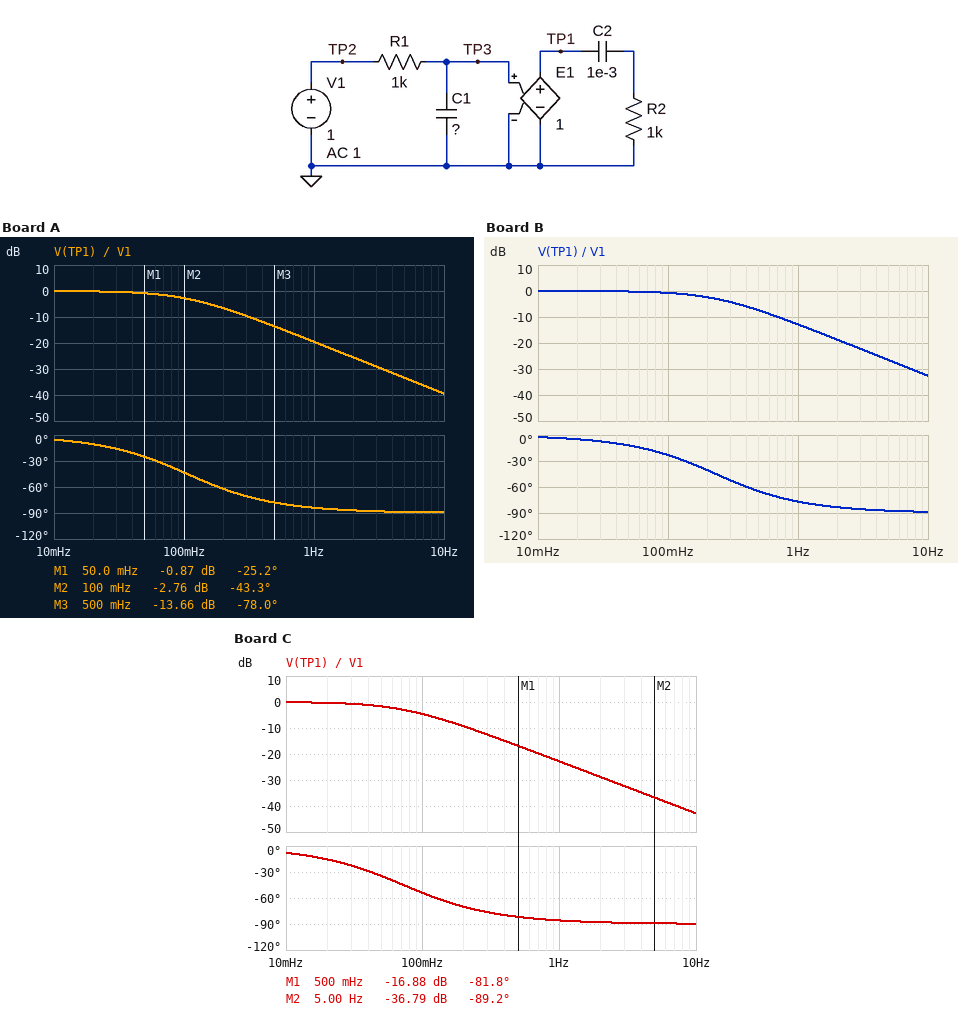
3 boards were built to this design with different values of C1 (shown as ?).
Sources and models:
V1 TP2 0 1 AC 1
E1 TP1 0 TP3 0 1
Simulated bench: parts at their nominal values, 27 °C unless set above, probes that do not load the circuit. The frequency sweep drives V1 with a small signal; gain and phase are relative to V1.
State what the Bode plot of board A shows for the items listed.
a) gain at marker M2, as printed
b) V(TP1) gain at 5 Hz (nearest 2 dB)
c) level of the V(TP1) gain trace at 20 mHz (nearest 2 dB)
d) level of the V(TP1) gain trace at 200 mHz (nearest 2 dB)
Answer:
-2.76 dB
-34 dB
0 dB
-6 dB
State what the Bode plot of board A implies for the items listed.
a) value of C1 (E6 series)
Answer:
1.5 mF
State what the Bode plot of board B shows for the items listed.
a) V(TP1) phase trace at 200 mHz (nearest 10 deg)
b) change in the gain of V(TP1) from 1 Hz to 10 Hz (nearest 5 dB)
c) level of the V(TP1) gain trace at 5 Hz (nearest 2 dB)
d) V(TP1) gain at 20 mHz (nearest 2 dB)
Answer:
-40 deg
-20 dB
-26 dB
0 dB
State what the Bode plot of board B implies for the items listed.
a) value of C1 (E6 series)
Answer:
680 µF
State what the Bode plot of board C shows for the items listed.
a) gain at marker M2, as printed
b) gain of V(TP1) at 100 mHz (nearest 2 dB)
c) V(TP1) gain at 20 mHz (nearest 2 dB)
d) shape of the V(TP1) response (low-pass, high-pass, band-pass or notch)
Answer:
-36.79 dB
-4 dB
0 dB
low-pass
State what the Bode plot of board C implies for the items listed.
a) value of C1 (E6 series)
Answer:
2.2 mF
